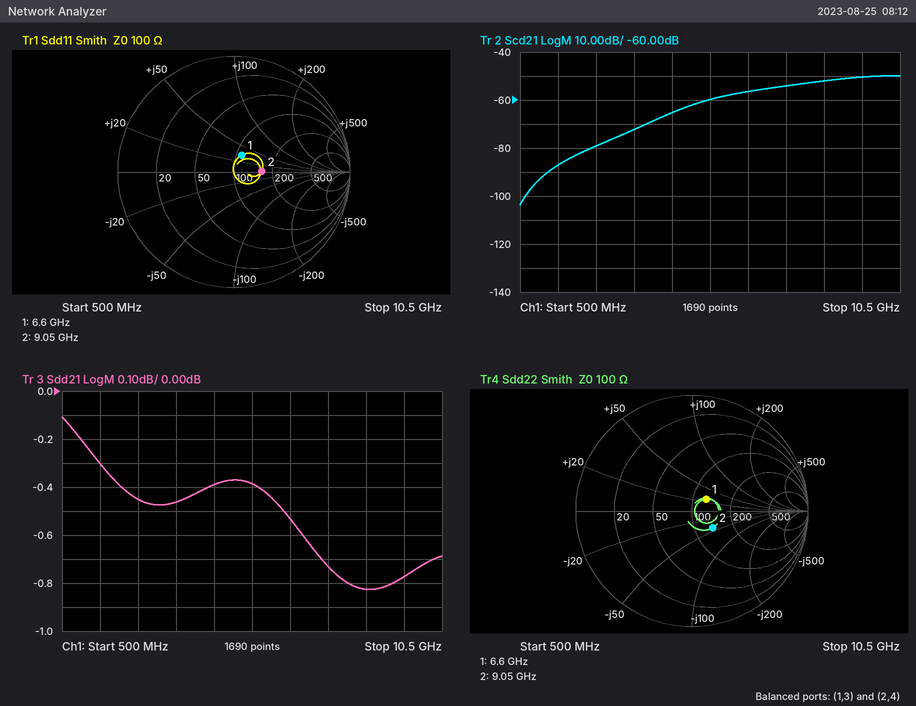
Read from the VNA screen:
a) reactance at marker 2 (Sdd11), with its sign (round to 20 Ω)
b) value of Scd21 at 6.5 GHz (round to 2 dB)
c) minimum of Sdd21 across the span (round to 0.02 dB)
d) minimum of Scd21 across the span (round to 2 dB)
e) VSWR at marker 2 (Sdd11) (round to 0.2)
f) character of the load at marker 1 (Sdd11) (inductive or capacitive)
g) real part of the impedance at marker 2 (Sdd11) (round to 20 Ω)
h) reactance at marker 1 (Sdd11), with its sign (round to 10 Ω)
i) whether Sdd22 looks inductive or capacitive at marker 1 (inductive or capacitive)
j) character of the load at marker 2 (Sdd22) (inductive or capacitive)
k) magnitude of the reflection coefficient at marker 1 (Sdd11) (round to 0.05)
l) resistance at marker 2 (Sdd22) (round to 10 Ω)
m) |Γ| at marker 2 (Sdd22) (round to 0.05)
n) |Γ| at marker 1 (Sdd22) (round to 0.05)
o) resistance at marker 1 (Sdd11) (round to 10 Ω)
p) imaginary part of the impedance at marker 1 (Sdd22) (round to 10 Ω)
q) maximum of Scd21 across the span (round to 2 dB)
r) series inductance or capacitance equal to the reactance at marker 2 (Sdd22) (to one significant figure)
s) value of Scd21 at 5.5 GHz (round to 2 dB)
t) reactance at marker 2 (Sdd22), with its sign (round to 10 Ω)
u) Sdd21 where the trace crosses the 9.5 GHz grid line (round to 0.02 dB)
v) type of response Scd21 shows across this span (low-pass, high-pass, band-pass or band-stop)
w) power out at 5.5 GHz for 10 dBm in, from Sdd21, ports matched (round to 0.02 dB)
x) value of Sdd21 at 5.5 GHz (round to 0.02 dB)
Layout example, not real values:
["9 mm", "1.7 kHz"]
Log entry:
["0 Ω", "-56 dB", "-0.82 dB", "-104 dB", "1.6", "inductive", "160 Ω", "+30 Ω", "inductive", "capacitive", "0.15", "140 Ω", "0.25", "0.15", "110 Ω", "+30 Ω", "-50 dB", "400 fF", "-60 dB", "-40 Ω", "-0.78 dB", "high-pass", "9.62 dBm", "-0.38 dB"]
